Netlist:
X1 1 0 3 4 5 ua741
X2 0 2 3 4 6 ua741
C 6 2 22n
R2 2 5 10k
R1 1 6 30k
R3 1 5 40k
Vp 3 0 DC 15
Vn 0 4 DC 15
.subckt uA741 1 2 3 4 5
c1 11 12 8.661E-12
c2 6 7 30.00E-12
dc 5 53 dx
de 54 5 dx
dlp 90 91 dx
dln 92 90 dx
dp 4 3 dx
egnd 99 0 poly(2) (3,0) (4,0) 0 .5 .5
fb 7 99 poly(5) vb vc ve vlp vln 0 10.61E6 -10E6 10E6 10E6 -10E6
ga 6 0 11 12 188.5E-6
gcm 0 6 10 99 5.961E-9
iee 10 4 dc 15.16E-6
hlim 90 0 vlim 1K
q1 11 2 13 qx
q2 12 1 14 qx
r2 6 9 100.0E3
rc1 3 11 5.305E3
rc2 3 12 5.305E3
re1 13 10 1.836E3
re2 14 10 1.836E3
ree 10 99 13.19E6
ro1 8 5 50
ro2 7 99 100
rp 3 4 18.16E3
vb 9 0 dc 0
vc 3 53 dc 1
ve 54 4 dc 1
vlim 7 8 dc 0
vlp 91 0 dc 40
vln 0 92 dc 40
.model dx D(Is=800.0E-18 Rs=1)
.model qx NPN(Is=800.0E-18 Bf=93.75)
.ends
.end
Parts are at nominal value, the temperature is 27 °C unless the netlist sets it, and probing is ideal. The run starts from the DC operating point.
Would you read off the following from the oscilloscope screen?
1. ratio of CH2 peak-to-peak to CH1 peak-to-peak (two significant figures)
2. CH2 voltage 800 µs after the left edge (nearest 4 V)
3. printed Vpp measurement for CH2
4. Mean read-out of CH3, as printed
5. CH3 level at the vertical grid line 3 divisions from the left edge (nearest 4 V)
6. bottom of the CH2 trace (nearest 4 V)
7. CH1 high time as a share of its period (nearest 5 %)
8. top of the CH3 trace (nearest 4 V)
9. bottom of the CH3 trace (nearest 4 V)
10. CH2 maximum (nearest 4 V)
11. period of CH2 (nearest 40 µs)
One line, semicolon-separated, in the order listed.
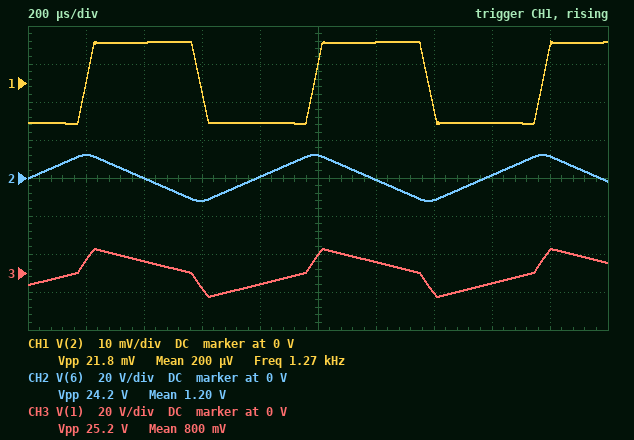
1100; 0 V; 24.2 V; 800 mV; -8 V; -12 V; 50 %; 12 V; -12 V; 12 V; 800 µs
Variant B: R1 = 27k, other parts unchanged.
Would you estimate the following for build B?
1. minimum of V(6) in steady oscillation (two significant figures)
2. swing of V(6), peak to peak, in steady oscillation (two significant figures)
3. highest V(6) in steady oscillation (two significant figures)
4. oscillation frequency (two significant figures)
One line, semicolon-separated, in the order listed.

-11 V; 22 V; 11 V; 1.4 kHz
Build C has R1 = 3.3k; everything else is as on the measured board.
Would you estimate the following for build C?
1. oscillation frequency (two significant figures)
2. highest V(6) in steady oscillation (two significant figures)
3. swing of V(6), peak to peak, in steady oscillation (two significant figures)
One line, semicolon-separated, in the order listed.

5.0 kHz; 2.3 V; 4.7 V
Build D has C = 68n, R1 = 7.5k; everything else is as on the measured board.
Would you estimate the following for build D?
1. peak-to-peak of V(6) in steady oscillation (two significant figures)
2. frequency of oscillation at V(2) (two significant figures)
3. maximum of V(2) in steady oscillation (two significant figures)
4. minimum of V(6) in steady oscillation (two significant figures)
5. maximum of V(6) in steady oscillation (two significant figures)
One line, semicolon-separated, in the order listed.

6.2 V; 1.6 kHz; 3.9 mV; -3.1 V; 3.1 V
